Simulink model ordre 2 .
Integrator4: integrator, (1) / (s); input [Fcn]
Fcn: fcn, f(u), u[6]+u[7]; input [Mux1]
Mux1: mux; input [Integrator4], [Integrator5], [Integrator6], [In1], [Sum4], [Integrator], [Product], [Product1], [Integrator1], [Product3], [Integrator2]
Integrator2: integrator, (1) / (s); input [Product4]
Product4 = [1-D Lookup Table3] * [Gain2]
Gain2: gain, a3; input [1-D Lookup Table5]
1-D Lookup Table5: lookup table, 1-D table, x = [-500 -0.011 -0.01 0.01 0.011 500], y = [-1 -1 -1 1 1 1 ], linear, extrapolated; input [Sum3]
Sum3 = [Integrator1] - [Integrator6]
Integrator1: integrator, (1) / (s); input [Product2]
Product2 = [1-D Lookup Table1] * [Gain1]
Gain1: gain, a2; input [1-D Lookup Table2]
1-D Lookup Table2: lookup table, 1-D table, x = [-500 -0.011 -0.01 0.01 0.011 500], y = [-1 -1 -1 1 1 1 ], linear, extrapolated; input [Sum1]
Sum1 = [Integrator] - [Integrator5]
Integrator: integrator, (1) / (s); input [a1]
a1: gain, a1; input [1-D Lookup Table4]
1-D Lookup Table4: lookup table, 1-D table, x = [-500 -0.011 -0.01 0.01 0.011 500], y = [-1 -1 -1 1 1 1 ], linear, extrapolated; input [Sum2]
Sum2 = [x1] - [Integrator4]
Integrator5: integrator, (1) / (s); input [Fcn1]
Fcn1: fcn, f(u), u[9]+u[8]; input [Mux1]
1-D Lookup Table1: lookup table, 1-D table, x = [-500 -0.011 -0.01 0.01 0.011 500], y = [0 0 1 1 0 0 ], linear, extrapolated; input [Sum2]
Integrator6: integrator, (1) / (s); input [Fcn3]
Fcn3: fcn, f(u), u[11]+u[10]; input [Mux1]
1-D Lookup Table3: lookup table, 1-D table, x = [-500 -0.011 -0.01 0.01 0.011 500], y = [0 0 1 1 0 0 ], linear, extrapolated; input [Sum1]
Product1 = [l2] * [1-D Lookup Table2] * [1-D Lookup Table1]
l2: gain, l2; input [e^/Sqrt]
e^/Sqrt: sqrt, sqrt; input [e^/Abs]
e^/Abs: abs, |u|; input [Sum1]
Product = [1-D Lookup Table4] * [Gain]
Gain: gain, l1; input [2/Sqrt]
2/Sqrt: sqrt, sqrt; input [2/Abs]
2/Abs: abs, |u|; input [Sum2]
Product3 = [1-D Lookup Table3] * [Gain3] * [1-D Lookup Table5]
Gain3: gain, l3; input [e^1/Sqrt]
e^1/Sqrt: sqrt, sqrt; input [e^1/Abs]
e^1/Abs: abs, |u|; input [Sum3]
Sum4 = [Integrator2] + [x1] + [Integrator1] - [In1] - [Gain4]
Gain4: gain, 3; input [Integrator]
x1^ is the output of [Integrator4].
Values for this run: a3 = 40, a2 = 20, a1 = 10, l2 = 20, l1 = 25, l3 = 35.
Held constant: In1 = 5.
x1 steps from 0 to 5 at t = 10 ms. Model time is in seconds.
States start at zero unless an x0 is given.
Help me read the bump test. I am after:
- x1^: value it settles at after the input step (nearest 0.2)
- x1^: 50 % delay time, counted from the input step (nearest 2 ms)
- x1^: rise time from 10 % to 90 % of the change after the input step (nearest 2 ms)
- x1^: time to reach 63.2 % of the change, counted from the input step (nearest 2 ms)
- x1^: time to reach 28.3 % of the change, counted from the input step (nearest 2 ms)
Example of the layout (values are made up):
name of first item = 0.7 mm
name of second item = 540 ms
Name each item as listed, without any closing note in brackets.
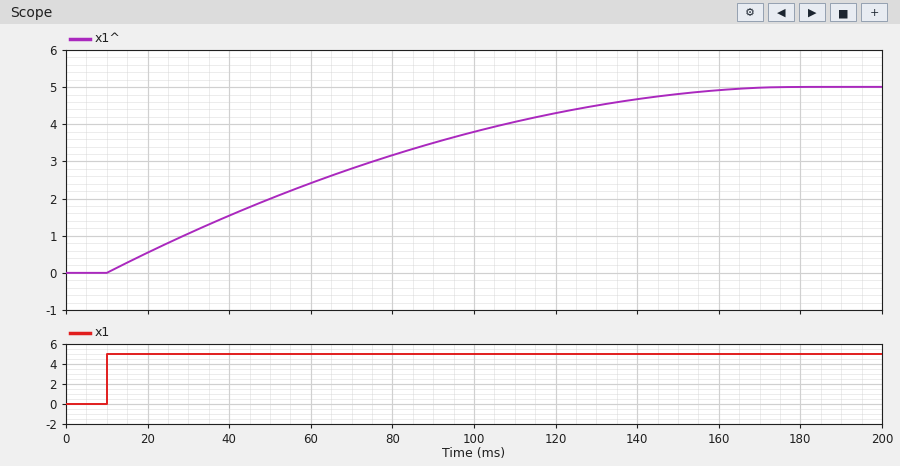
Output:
x1^: value it settles at after the input step = 5.0
x1^: 50 % delay time, counted from the input step = 52 ms
x1^: rise time from 10 % to 90 % of the change after the input step = 110 ms
x1^: time to reach 63.2 % of the change, counted from the input step = 70 ms
x1^: time to reach 28.3 % of the change, counted from the input step = 28 ms
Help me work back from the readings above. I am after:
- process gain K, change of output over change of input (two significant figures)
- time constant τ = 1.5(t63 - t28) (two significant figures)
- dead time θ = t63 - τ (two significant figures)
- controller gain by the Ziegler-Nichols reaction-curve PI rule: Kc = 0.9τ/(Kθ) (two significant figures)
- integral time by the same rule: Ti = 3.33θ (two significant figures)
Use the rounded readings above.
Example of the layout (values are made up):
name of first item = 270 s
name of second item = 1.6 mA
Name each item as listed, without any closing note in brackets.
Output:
process gain K, change of output over change of input = 1.0
time constant τ = 1.5(t63 - t28) = 63 ms
dead time θ = t63 - τ = 7.0 ms
controller gain by the Ziegler-Nichols reaction-curve PI rule: Kc = 0.9τ/(Kθ) = 8.1
integral time by the same rule: Ti = 3.33θ = 23 ms
